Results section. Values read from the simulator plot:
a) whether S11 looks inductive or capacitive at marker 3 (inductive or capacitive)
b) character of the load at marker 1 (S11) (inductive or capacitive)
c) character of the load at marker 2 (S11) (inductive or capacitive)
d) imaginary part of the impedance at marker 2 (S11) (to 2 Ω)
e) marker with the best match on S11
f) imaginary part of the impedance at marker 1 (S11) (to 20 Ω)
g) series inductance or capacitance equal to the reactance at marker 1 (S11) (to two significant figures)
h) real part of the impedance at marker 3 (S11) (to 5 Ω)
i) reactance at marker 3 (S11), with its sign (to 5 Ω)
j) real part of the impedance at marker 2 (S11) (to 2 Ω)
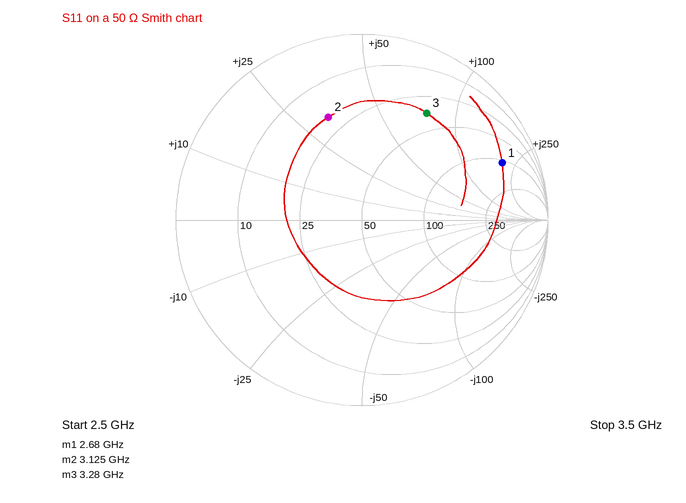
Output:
inductive
inductive
inductive
+32 Ω
marker 2
+200 Ω
12 nH
35 Ω
+75 Ω
20 Ω
